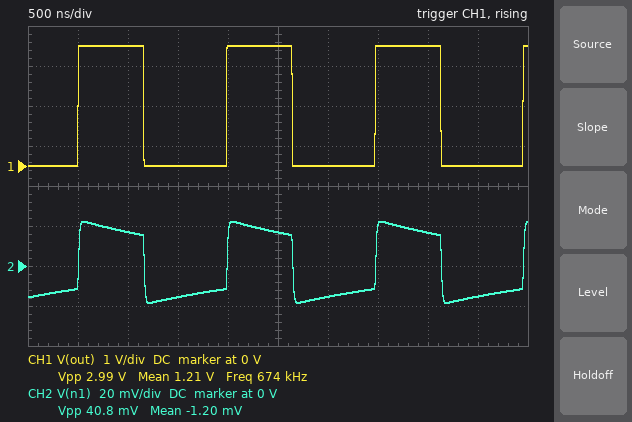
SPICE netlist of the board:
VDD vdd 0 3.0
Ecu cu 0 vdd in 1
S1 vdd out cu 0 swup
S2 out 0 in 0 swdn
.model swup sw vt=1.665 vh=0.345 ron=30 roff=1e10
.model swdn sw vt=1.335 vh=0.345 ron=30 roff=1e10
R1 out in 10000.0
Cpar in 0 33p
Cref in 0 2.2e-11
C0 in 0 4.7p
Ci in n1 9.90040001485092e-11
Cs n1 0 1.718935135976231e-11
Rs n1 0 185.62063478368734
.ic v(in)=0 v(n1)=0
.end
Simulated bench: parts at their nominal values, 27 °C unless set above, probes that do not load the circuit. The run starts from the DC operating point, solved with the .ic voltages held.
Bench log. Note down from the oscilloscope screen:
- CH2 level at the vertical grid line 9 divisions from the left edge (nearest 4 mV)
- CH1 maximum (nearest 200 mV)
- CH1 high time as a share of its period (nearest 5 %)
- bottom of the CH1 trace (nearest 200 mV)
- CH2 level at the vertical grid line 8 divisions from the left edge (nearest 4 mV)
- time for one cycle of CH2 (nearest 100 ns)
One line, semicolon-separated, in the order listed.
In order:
-16 mV; 3.0 V; 45 %; 0 V; 16 mV; 1.5 µs
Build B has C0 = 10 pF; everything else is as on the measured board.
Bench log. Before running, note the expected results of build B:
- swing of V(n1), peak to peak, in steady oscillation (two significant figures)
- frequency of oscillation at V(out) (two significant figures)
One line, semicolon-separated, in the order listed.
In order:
39 mV; 650 kHz
